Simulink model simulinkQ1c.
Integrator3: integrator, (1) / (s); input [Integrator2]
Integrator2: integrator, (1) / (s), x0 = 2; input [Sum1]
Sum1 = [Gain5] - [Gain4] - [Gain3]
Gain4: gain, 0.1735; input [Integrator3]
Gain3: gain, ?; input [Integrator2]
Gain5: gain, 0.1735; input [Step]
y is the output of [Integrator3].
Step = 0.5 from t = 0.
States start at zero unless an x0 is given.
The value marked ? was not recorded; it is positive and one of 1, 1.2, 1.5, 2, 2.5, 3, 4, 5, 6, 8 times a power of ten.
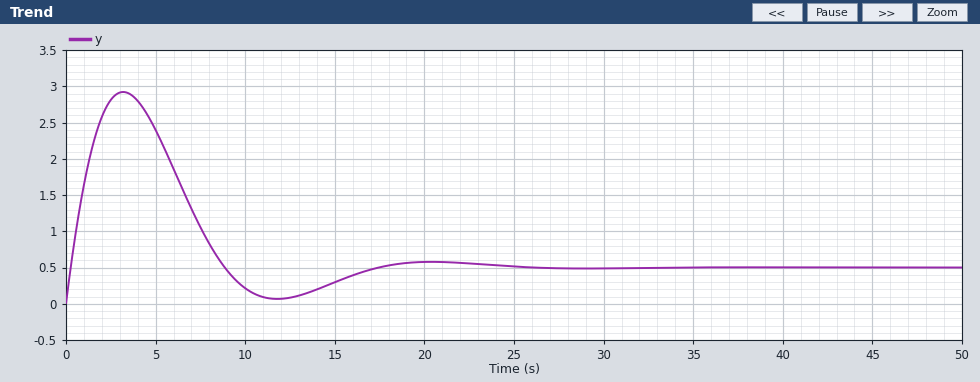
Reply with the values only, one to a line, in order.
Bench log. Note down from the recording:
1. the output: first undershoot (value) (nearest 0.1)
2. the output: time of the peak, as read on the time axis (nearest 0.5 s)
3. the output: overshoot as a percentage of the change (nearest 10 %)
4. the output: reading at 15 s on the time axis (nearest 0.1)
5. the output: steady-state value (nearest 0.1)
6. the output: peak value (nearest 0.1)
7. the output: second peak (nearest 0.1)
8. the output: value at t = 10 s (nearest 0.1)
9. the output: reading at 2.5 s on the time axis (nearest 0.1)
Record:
0.1
3.0 s
480 %
0.3
0.5
2.9
0.6
0.2
2.8
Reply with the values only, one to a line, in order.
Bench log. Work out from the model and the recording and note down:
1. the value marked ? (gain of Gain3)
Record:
0.4
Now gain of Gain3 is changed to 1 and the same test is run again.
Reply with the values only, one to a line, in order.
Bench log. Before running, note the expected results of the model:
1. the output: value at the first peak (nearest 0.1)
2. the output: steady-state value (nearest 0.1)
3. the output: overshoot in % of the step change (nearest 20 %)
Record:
1.7
0.5
240 %
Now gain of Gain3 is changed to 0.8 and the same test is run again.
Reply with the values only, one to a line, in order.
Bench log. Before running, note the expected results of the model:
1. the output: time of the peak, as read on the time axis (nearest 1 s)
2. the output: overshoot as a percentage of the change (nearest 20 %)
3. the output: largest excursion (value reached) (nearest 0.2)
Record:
3 s
300 %
2.0
